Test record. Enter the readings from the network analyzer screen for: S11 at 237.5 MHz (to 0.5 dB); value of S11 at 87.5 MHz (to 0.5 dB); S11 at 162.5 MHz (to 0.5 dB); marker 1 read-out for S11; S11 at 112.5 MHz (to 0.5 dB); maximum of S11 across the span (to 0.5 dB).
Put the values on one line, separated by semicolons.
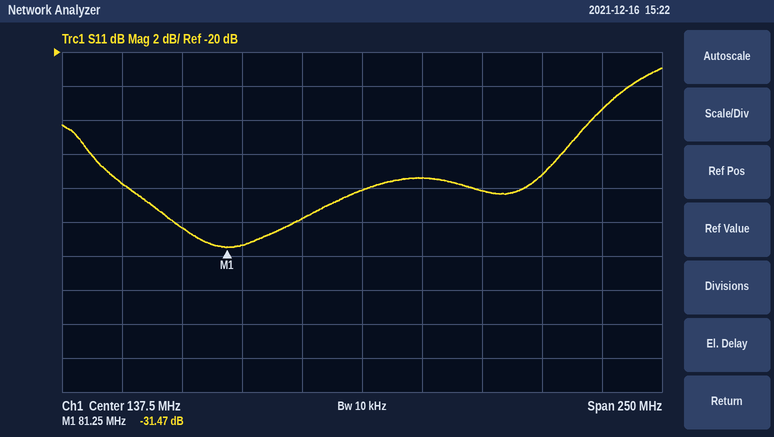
-23.5 dB; -31.5 dB; -27.5 dB; -31.47 dB; -30.0 dB; -21.0 dB
